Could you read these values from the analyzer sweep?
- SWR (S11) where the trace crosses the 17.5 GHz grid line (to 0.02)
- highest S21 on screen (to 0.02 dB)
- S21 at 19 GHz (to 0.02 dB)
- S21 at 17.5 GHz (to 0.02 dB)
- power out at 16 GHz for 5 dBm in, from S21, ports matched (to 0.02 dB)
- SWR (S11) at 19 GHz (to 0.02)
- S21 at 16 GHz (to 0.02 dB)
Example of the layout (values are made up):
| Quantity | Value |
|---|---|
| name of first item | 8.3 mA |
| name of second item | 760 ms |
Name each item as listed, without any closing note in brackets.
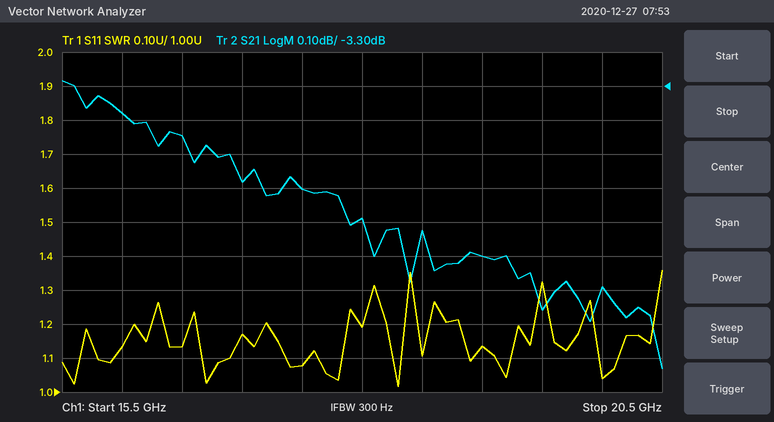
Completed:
| Quantity | Value |
|---|---|
| SWR (S11) where the trace crosses the 17.5 GHz grid line | 1.08 |
| highest S21 on screen | -3.28 dB |
| S21 at 19 GHz | -3.80 dB |
| S21 at 17.5 GHz | -3.60 dB |
| power out at 16 GHz for 5 dBm in, from S21, ports matched | 1.62 dBm |
| SWR (S11) at 19 GHz | 1.14 |
| S21 at 16 GHz | -3.38 dB |
